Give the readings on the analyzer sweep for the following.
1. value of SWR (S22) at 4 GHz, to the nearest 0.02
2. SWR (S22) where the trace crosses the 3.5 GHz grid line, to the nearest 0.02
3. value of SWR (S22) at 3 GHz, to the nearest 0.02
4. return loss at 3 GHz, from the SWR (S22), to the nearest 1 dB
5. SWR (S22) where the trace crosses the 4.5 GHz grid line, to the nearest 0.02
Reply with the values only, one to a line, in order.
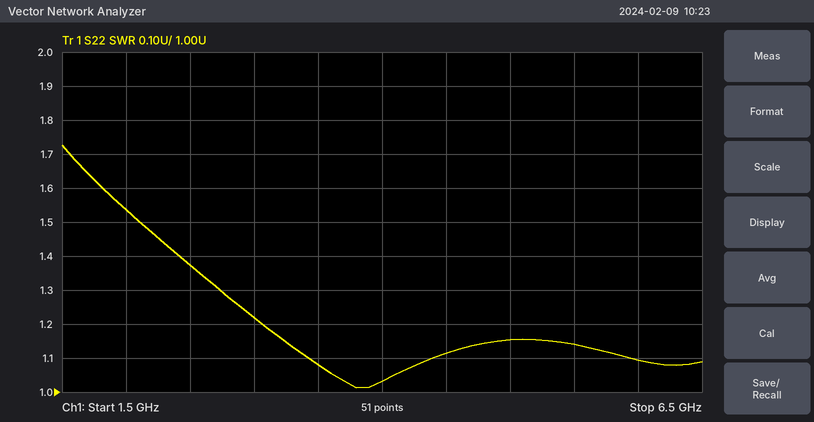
1.04
1.08
1.22
20 dB
1.12
